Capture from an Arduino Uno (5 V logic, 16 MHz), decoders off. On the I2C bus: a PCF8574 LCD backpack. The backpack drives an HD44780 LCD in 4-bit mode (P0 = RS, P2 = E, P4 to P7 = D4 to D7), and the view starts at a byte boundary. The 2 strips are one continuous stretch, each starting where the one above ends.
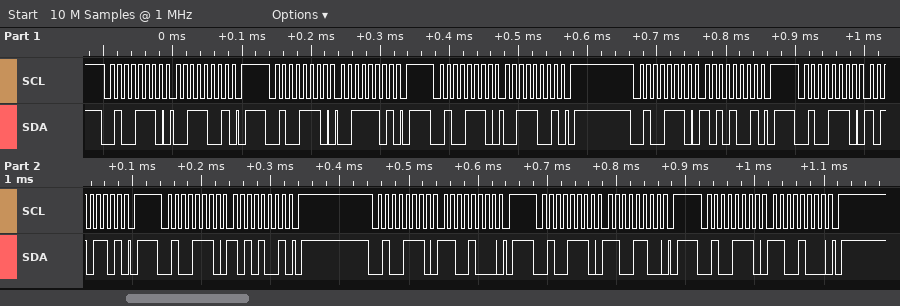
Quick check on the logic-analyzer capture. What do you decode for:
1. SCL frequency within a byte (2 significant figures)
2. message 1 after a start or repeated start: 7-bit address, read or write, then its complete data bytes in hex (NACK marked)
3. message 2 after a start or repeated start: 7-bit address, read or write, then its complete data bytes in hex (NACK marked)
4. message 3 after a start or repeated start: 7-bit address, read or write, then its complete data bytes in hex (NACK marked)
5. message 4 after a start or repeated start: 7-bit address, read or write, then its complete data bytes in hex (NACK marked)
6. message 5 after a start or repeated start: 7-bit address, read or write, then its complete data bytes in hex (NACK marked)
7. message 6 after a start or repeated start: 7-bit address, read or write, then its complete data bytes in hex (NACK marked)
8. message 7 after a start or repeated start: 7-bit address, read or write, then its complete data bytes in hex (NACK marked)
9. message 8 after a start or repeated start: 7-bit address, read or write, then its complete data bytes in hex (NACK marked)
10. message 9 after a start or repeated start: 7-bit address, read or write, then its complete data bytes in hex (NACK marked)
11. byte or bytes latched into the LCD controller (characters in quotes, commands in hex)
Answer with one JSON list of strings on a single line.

["100 kHz", "0x27 write: 39", "0x27 write: 3D", "0x27 write: 39", "0x27 write: A9", "0x27 write: AD", "0x27 write: A9", "0x27 write: C8", "0x27 write: CC", "0x27 write: C8", "':'"]
